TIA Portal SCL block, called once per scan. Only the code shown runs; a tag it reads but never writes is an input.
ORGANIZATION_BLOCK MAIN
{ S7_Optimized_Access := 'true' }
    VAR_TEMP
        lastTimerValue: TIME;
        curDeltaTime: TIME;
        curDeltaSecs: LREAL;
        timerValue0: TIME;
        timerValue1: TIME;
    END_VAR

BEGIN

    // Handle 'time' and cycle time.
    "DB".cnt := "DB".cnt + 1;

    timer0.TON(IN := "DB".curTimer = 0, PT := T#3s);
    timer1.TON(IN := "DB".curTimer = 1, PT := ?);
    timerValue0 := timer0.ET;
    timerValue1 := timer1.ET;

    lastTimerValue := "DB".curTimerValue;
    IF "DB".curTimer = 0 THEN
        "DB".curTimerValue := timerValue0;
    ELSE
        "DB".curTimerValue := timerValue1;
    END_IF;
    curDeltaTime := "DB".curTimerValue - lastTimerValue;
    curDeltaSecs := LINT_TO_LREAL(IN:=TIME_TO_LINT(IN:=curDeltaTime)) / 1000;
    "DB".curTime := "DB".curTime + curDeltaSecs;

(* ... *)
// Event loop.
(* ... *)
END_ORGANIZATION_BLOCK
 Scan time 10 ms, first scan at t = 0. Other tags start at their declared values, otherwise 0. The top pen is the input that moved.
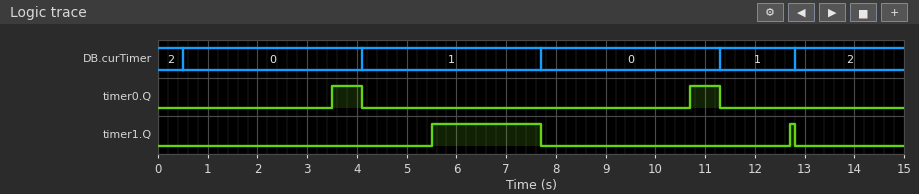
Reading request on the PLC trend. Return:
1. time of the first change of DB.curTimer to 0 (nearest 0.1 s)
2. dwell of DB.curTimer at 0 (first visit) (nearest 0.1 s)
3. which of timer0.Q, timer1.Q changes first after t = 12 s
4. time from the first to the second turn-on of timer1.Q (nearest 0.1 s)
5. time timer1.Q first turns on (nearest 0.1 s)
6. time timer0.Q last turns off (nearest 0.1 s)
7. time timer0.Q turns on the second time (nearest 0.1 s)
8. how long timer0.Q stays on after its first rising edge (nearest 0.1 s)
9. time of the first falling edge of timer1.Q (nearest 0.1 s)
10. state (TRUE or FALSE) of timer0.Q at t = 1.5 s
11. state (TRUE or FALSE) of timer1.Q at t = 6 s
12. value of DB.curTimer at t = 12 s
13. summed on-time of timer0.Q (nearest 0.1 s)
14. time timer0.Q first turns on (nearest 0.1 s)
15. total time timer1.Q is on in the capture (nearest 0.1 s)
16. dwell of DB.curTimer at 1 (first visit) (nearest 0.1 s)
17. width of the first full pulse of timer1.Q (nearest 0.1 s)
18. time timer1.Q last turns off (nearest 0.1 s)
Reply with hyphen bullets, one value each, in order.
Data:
- 0.5 s
- 3.6 s
- timer1.Q
- 7.2 s
- 5.5 s
- 11.3 s
- 10.7 s
- 0.6 s
- 7.7 s
- FALSE
- TRUE
- 1
- 1.2 s
- 3.5 s
- 2.3 s
- 3.6 s
- 2.2 s
- 12.8 s
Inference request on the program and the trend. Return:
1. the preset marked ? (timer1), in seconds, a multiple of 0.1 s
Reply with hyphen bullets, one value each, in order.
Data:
- 1.4 s
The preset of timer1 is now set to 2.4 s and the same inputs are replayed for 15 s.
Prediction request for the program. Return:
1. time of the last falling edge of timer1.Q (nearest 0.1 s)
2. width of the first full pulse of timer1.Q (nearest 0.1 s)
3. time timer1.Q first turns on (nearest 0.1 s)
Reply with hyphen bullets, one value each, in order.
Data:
- 7.7 s
- 1.2 s
- 6.5 s
